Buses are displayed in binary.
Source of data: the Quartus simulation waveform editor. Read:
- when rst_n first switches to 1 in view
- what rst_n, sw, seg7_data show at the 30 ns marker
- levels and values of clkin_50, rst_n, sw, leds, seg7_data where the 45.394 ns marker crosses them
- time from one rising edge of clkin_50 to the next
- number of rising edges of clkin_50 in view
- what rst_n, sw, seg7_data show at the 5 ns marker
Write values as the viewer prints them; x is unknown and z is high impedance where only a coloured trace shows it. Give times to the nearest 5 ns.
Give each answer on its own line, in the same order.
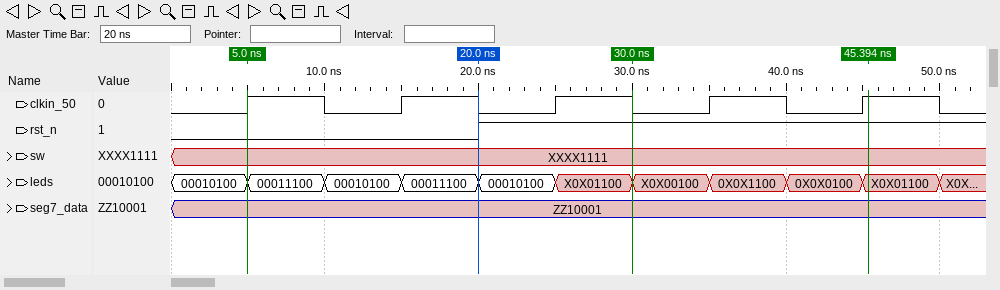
20 ns
rst_n=1, sw=XXXX1111, seg7_data=ZZ10001
clkin_50=1, rst_n=1, sw=XXXX1111, leds=X0X01100, seg7_data=ZZ10001
10 ns
5
rst_n=0, sw=XXXX1111, seg7_data=ZZ10001
